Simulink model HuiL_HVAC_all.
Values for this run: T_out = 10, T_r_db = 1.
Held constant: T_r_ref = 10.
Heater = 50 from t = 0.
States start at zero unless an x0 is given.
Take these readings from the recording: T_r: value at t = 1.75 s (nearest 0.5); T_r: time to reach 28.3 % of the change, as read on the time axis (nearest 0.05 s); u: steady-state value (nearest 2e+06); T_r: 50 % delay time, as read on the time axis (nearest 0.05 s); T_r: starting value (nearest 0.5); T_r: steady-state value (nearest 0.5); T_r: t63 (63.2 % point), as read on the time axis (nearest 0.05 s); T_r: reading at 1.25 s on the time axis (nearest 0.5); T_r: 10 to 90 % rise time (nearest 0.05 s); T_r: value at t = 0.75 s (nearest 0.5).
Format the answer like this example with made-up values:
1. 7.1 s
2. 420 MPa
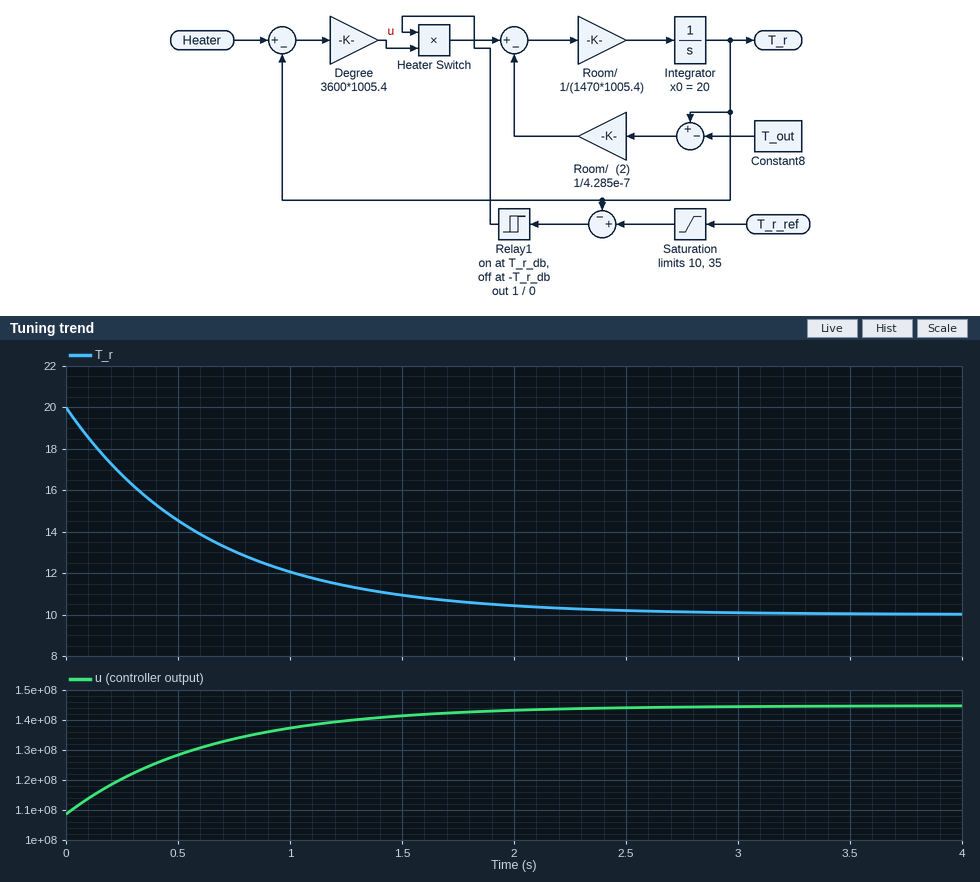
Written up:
1. 10.5
2. 0.20 s
3. 144000000
4. 0.45 s
5. 20.0
6. 10.0
7. 0.65 s
8. 11.5
9. 1.40 s
10. 13.0
